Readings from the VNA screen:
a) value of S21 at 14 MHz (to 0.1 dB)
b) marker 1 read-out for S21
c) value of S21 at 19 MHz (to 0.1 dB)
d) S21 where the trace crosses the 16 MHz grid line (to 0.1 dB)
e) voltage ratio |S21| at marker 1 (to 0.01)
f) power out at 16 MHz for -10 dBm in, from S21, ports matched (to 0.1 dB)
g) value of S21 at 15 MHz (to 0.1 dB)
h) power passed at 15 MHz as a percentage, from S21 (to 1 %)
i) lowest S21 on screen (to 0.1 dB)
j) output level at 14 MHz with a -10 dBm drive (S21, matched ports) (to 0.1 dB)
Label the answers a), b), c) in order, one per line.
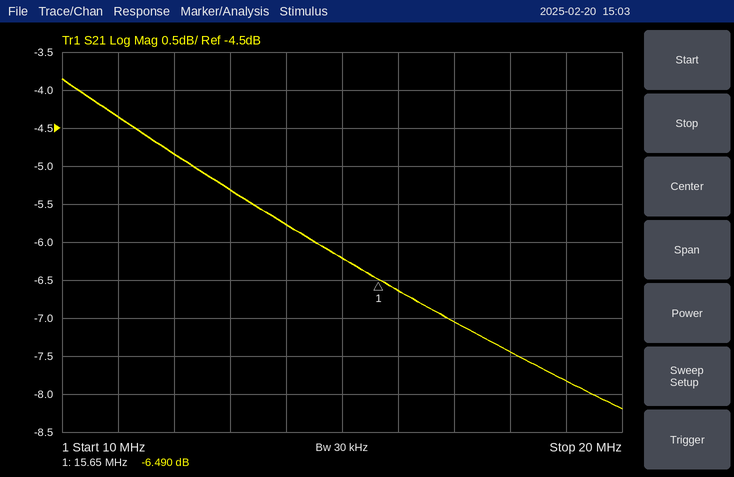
a) -5.8 dB
b) -6.490 dB
c) -7.8 dB
d) -6.6 dB
e) 0.47
f) -16.6 dBm
g) -6.2 dB
h) 24 %
i) -8.2 dB
j) -15.8 dBm
